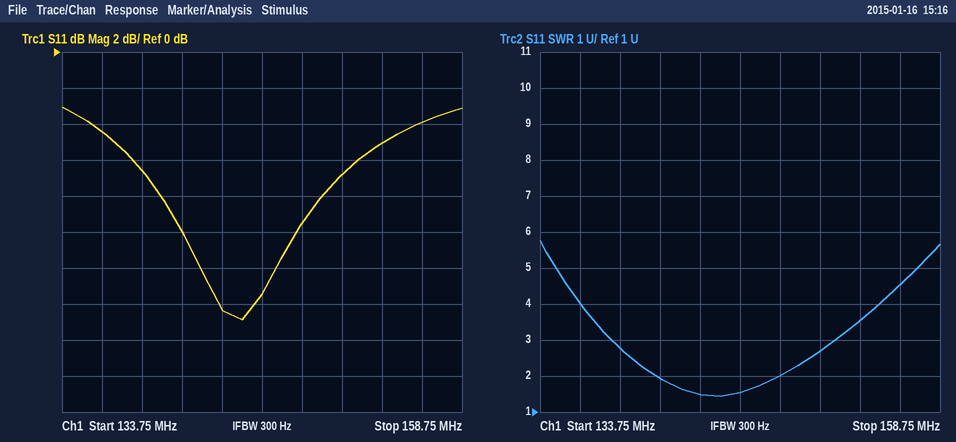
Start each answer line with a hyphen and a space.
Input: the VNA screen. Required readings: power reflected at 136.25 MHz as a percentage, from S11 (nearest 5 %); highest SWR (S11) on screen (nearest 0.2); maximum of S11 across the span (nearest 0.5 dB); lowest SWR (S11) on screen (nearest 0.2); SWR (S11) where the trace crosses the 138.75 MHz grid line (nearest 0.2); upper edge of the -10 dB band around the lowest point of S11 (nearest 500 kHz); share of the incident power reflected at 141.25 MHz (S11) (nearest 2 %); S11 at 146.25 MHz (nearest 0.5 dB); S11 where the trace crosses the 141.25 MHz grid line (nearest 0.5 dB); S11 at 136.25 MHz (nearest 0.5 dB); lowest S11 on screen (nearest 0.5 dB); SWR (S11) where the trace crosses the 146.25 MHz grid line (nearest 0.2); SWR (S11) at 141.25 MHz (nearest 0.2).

- 35 %
- 5.8
- -3.0 dB
- 1.4
- 2.8
- 148.5 MHz
- 10 %
- -13.5 dB
- -10.0 dB
- -4.5 dB
- -15.0 dB
- 1.6
- 2.0
